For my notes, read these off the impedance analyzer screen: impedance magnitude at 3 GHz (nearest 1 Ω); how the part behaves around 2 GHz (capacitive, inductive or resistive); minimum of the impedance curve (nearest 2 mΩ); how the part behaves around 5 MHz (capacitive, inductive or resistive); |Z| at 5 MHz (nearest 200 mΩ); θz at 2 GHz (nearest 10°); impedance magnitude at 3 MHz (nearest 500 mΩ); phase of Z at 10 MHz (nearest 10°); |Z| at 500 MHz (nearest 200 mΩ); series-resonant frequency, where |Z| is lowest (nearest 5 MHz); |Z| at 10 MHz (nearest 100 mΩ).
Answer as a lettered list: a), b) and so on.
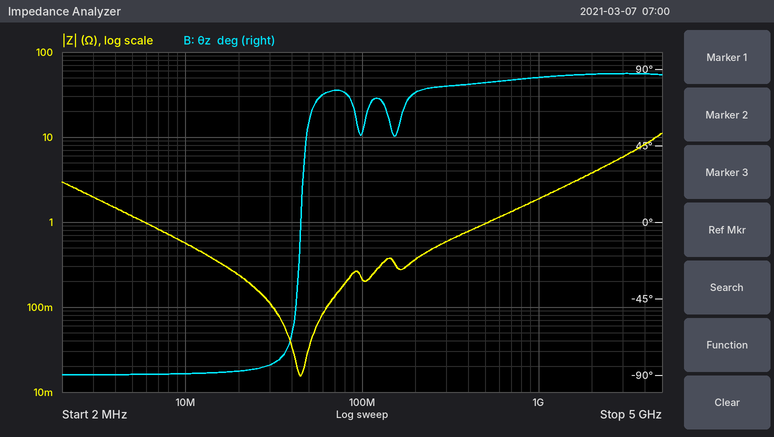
a) 6 Ω
b) inductive
c) 16 mΩ
d) capacitive
e) 1.2 Ω
f) 90°
g) 2.0 Ω
h) -90°
i) 1.0 Ω
j) 45 MHz
k) 600 mΩ
